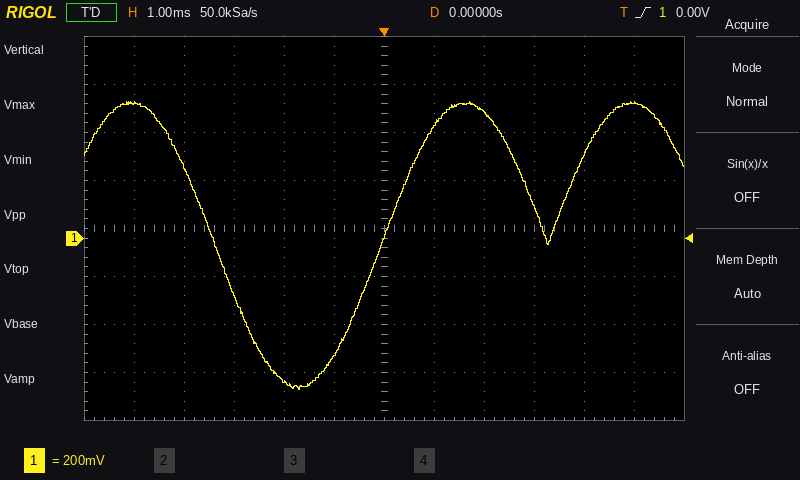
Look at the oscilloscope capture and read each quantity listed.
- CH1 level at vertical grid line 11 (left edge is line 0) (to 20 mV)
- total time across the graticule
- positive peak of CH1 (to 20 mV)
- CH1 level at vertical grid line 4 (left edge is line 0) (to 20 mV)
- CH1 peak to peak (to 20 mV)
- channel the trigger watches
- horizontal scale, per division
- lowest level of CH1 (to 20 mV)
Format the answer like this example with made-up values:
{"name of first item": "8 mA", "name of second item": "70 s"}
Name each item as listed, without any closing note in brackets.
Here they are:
{"CH1 level at vertical grid line 11 (left edge is line 0)": "560 mV", "total time across the graticule": "12 ms", "positive peak of CH1": "560 mV", "CH1 level at vertical grid line 4 (left edge is line 0)": "-600 mV", "CH1 peak to peak": "1.20 V", "channel the trigger watches": "CH1", "horizontal scale, per division": "1 ms", "lowest level of CH1": "-640 mV"}
